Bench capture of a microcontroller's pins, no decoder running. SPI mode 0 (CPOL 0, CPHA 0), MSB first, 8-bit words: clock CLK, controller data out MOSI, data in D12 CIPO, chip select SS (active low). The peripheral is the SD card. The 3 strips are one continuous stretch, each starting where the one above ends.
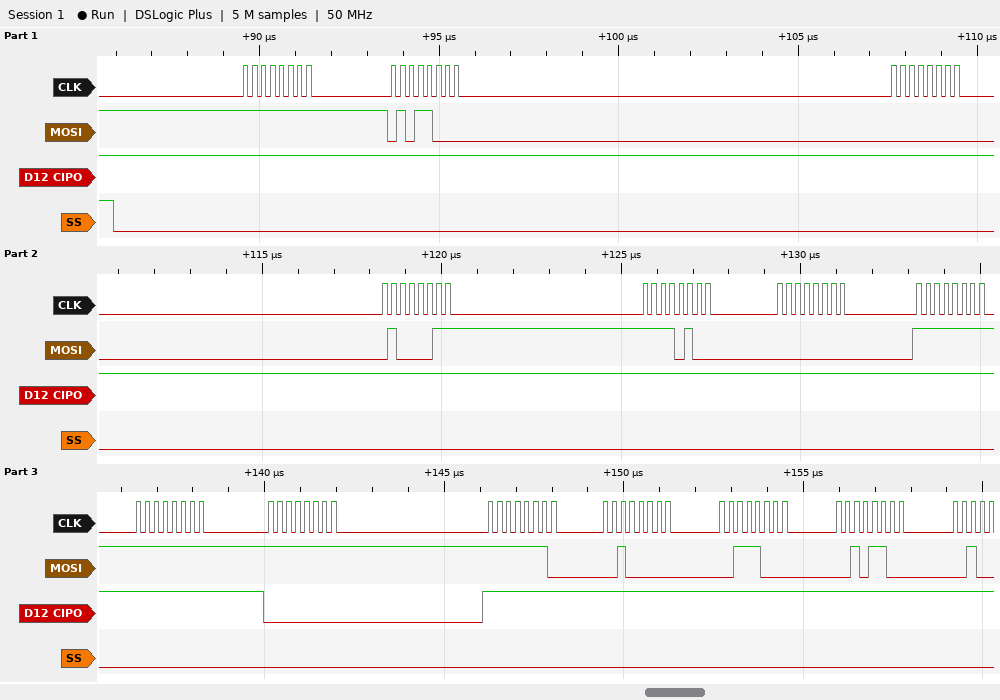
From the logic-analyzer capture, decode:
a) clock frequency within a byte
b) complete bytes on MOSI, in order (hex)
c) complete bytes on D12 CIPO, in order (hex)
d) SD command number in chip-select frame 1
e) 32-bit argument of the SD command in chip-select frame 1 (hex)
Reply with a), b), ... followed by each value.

a) 4 MHz
b) FF 58 00 43 F4 00 FF FF FF FE 20 38 2C
c) FF FF FF FF FF FF FF FF 00 FF FF FF FF
d) CMD24
e) 0x0043F400
